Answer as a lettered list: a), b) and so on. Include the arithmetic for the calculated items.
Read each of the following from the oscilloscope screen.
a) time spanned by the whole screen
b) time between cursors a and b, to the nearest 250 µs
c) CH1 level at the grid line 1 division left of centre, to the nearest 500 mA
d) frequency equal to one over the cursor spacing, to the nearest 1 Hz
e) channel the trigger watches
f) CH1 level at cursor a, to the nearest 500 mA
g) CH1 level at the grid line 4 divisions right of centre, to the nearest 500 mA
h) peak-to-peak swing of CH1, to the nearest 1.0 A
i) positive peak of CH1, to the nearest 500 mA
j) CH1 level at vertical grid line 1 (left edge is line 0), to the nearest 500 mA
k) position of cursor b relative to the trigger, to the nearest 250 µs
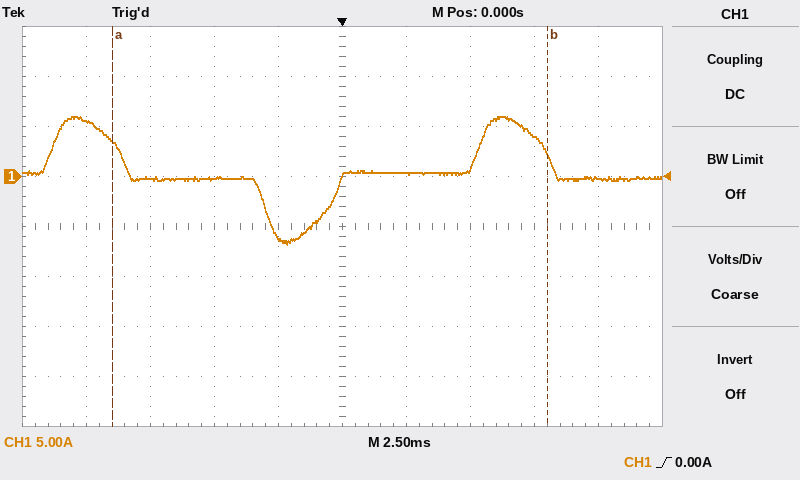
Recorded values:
a) 25 ms
b) 17.00 ms
c) -6.0 A
d) 1 / 17.00 ms ≈ 59 Hz
e) CH1
f) 3.5 A
g) 0.0 A
h) 13.0 A
i) 6.0 A
j) 5.5 A
k) +8.00 ms
